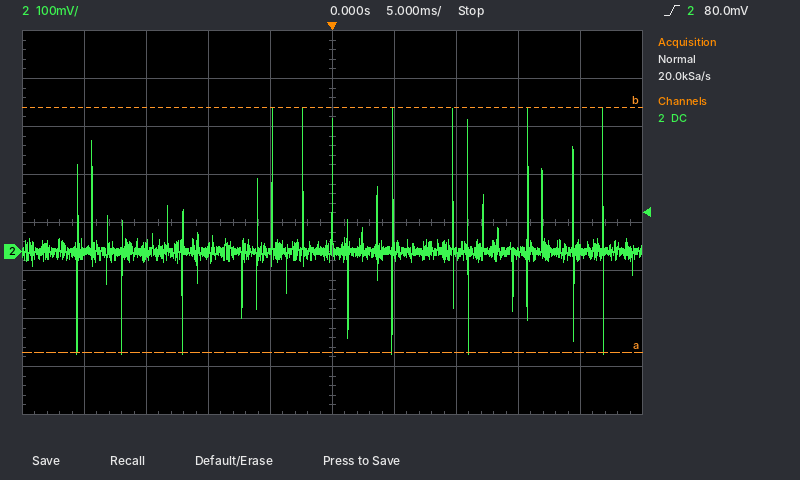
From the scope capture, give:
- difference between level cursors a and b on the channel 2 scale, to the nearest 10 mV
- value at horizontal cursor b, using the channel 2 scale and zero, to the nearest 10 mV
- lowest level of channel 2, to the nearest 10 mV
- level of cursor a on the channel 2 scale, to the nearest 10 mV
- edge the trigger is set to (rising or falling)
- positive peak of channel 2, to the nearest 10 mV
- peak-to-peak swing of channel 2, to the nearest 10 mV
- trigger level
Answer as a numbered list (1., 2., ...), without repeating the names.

1. 510 mV
2. 300 mV
3. -210 mV
4. -210 mV
5. rising
6. 300 mV
7. 510 mV
8. 80.0 mV
